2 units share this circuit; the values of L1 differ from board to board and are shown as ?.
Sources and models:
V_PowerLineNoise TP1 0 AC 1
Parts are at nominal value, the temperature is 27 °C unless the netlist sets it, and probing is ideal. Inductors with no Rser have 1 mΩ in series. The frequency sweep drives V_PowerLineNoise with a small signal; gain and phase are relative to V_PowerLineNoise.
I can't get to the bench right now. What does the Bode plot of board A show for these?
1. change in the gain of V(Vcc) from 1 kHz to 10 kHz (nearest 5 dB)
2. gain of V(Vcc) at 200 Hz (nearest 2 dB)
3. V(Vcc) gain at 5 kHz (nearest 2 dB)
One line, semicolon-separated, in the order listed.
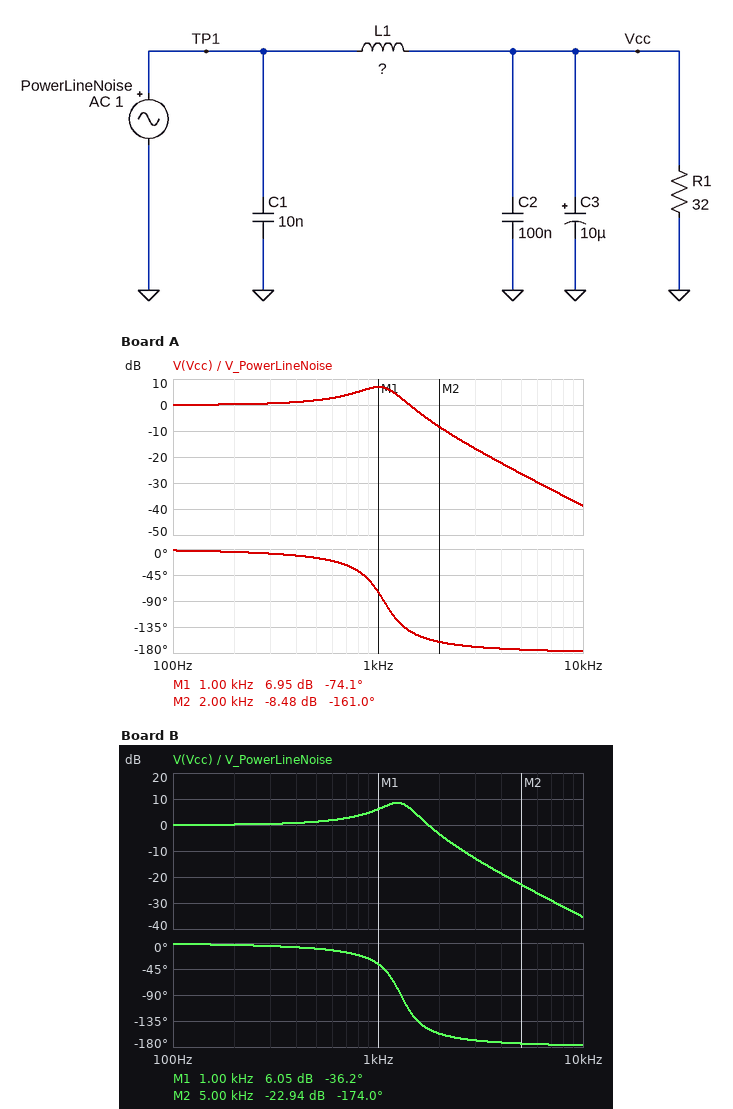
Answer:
-45 dB; 0 dB; -26 dB
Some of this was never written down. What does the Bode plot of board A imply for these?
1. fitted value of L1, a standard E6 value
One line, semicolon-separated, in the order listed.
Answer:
2.2 mH
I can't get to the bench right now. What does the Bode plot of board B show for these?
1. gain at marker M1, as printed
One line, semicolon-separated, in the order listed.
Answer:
6.05 dB
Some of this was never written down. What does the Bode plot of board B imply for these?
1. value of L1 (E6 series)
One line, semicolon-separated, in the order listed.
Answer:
1.5 mH
